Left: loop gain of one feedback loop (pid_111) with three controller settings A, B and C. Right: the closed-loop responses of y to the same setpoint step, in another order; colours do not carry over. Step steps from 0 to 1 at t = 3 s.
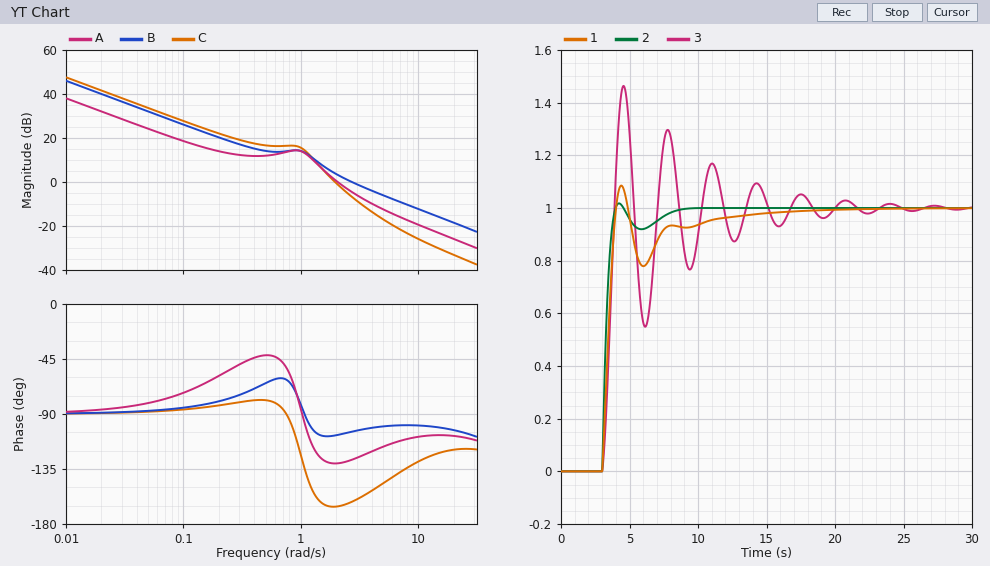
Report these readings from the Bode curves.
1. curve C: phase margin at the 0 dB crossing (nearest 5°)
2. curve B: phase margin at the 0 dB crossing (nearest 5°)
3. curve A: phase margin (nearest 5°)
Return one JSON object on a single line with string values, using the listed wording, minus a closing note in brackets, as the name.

{"curve C: phase margin at the 0 dB crossing": "15°", "curve B: phase margin at the 0 dB crossing": "75°", "curve A: phase margin": "50°"}
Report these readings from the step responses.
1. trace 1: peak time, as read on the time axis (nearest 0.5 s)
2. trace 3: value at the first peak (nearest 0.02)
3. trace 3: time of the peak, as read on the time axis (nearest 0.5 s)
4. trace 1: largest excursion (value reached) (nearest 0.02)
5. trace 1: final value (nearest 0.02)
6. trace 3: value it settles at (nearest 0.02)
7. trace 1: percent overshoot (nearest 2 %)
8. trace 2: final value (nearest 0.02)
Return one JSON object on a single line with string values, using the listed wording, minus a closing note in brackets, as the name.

{"trace 1: peak time, as read on the time axis": "4.5 s", "trace 3: value at the first peak": "1.46", "trace 3: time of the peak, as read on the time axis": "4.5 s", "trace 1: largest excursion (value reached)": "1.08", "trace 1: final value": "1.00", "trace 3: value it settles at": "1.00", "trace 1: percent overshoot": "8 %", "trace 2: final value": "1.00"}
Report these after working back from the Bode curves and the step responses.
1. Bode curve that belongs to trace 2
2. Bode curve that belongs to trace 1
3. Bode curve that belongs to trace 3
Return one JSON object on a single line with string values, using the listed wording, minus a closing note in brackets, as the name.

{"Bode curve that belongs to trace 2": "B", "Bode curve that belongs to trace 1": "A", "Bode curve that belongs to trace 3": "C"}
